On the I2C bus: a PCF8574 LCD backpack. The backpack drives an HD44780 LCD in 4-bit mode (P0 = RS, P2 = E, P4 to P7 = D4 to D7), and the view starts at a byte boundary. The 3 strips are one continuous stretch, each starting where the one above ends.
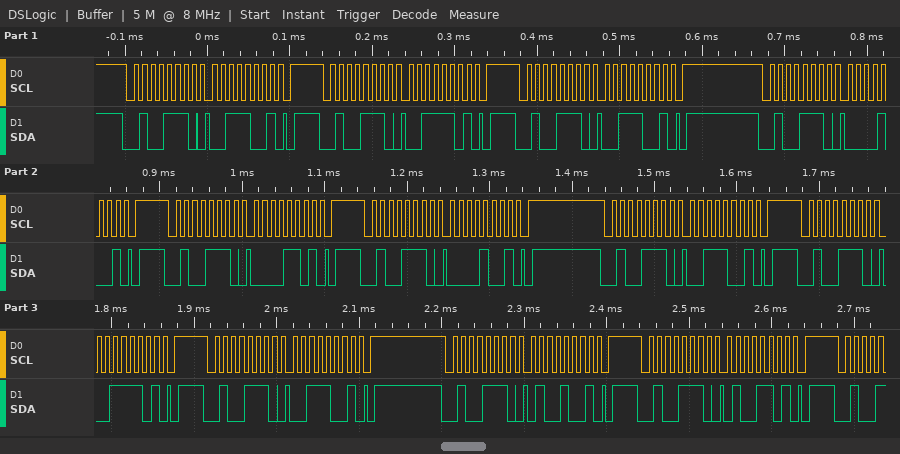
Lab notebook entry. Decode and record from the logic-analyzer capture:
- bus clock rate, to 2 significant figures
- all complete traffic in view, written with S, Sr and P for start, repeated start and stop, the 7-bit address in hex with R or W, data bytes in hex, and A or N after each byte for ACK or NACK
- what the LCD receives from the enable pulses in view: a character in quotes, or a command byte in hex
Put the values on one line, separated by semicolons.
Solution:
100 kHz; S 27W A 39 A P S 27W A 3D A P S 27W A 39 A P S 27W A 09 A P S 27W A 0D A P S 27W A 09 A P S 27W A 39 A P S 27W A 3D A P S 27W A 39 A P S 27W A 49 A P S 27W A 4D A P; '0'
